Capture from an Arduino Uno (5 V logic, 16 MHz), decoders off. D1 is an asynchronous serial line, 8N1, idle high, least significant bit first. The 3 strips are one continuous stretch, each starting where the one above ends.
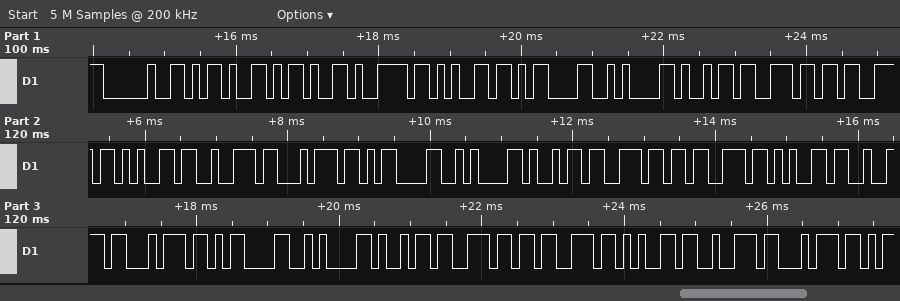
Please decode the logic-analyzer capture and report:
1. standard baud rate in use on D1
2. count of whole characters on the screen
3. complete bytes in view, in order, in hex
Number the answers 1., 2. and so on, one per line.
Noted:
1. 9600 baud
2. 29
3. 0x20 0x2D 0x2D 0x79 0x65 0x0D 0x0A 0x69 0x6E 0x73 0x65 0x72 0x74 0x0D 0x0A 0x69 0x6E 0x73 0x65 0x72 0x74 0x0D 0x0A 0x69 0x6E 0x73 0x65 0x72 0x74
